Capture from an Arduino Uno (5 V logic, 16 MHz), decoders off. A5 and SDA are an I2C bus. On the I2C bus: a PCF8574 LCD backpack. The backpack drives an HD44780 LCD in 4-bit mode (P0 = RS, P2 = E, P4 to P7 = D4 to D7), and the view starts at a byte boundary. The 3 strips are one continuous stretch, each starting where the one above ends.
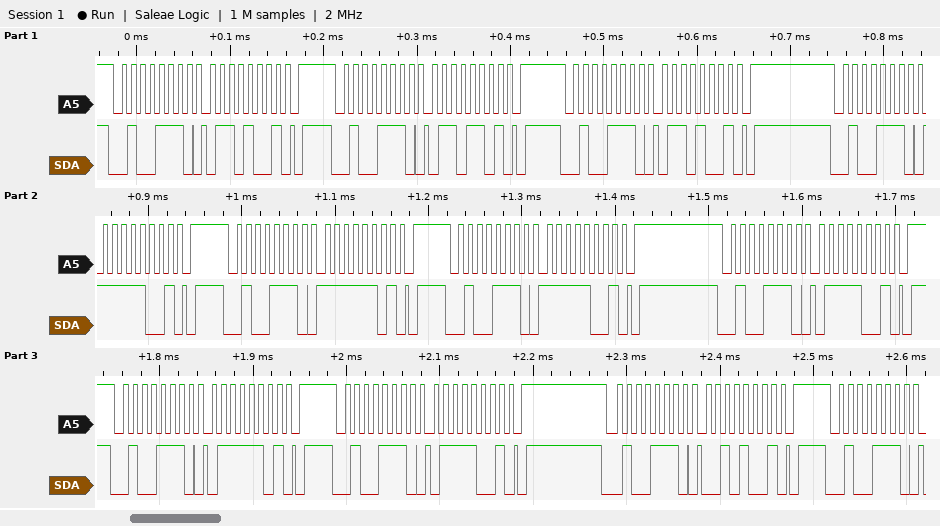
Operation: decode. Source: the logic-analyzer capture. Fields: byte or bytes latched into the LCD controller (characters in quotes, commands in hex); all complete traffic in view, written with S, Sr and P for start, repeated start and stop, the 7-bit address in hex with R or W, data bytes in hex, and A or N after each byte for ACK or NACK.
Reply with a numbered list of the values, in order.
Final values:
1. 'o'
2. S 27W A 69 A P S 27W A 6D A P S 27W A 69 A P S 27W A F9 A P S 27W A FD A P S 27W A F9 A P S 27W A 79 A P S 27W A 7D A P S 27W A 79 A P S 27W A 29 A P S 27W A
